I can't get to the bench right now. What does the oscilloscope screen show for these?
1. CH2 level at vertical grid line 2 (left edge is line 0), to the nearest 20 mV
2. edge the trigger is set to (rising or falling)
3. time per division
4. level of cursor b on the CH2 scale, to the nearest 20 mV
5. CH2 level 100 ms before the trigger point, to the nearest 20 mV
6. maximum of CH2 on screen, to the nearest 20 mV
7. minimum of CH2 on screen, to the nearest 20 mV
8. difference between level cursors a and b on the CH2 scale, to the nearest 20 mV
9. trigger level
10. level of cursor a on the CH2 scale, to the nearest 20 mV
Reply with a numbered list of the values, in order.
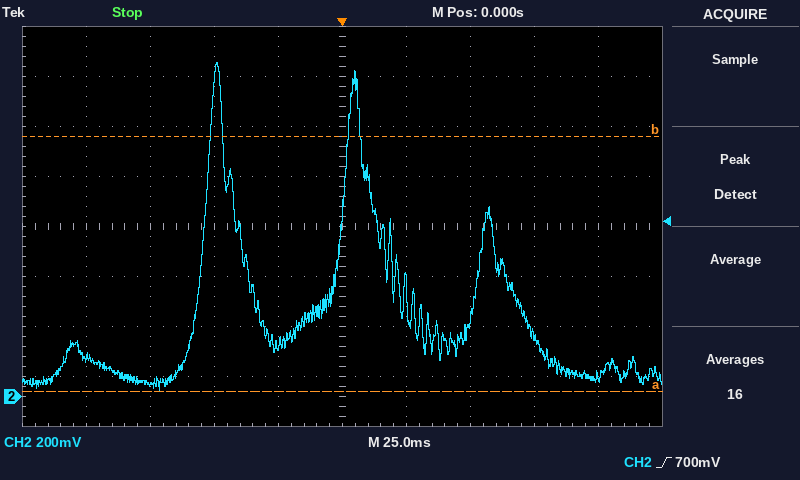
1. 40 mV
2. rising
3. 25 ms
4. 1.04 V
5. 160 mV
6. 1.34 V
7. 20 mV
8. 1.02 V
9. 700 mV
10. 20 mV
